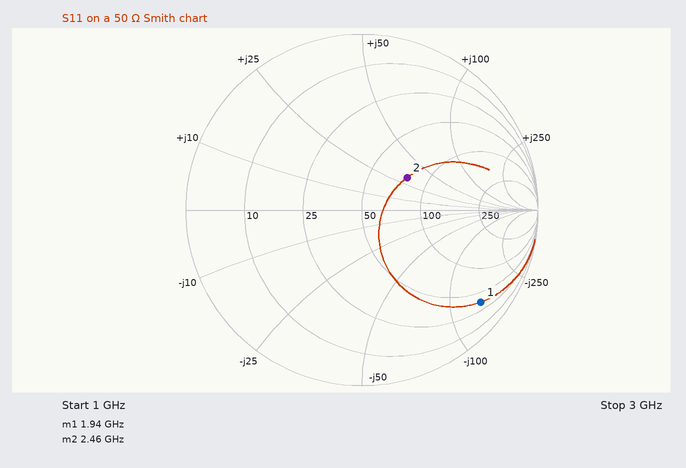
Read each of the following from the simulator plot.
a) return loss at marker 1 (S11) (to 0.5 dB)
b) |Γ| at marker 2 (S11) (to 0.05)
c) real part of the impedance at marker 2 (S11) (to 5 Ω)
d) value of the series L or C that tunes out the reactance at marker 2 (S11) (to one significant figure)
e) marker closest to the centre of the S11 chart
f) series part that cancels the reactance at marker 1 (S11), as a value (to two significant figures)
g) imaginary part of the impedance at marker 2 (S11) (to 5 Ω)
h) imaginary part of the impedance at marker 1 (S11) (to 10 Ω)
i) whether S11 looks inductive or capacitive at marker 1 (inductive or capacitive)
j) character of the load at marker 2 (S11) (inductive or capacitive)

1.5 dB
0.30
75 Ω
2 pF
marker 2
11 nH
+30 Ω
-140 Ω
capacitive
inductive
